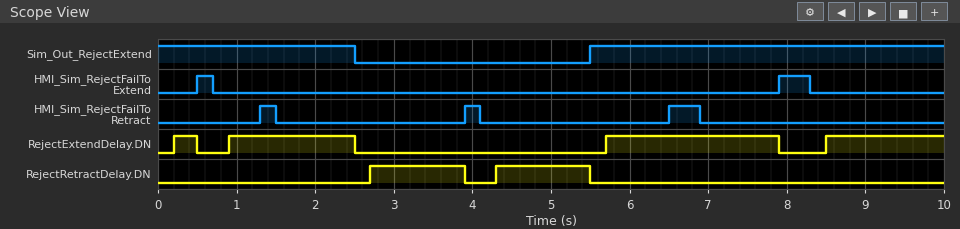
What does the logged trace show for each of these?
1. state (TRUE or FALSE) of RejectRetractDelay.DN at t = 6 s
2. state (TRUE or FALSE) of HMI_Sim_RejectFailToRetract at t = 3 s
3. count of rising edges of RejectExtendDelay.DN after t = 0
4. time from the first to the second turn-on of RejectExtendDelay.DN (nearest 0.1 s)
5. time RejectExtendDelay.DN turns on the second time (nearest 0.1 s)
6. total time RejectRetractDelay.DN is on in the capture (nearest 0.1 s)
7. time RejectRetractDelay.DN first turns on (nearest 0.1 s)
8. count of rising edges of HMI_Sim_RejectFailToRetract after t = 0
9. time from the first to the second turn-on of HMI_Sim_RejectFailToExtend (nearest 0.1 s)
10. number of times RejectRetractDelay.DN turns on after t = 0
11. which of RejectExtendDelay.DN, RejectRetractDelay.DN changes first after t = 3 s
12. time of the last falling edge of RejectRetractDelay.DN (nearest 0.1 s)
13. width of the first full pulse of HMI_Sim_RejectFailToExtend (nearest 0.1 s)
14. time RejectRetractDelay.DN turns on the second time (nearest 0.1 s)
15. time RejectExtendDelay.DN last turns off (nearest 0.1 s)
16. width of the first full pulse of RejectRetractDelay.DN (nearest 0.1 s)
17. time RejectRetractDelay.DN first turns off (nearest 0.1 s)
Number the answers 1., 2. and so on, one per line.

1. FALSE
2. FALSE
3. 4
4. 0.7 s
5. 0.9 s
6. 2.4 s
7. 2.7 s
8. 3
9. 7.4 s
10. 2
11. RejectRetractDelay.DN
12. 5.5 s
13. 0.2 s
14. 4.3 s
15. 7.9 s
16. 1.2 s
17. 3.9 s
